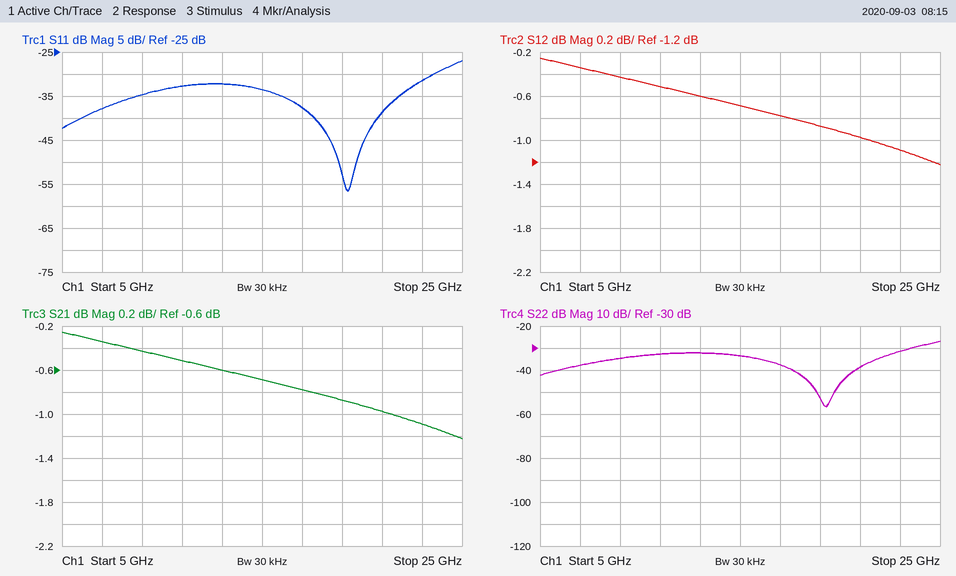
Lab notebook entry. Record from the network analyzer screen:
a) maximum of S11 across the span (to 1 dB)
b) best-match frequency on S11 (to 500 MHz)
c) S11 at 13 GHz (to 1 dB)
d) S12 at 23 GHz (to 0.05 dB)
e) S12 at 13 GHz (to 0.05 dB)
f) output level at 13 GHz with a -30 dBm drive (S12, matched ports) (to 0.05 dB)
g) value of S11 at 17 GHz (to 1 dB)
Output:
-27 dB
19.5 GHz
-32 dB
-1.10 dB
-0.60 dB
-30.60 dBm
-38 dB
